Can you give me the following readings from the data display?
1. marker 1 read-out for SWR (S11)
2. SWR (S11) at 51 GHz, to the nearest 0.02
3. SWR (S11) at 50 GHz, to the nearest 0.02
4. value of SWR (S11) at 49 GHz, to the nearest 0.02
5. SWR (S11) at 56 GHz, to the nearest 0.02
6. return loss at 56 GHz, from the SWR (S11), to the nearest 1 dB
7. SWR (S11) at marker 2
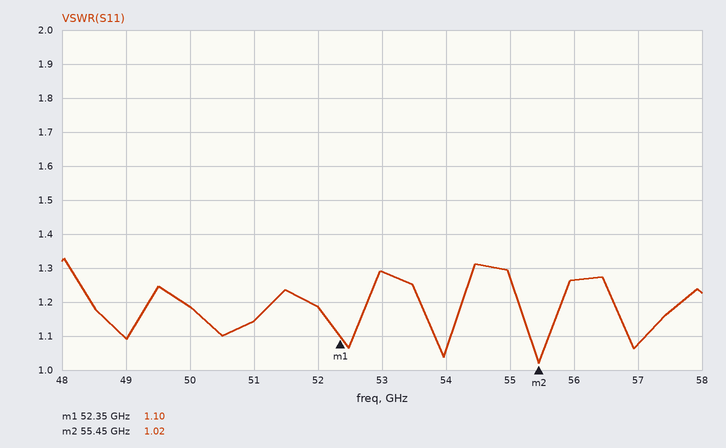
1.10
1.14
1.18
1.10
1.26
19 dB
1.02
